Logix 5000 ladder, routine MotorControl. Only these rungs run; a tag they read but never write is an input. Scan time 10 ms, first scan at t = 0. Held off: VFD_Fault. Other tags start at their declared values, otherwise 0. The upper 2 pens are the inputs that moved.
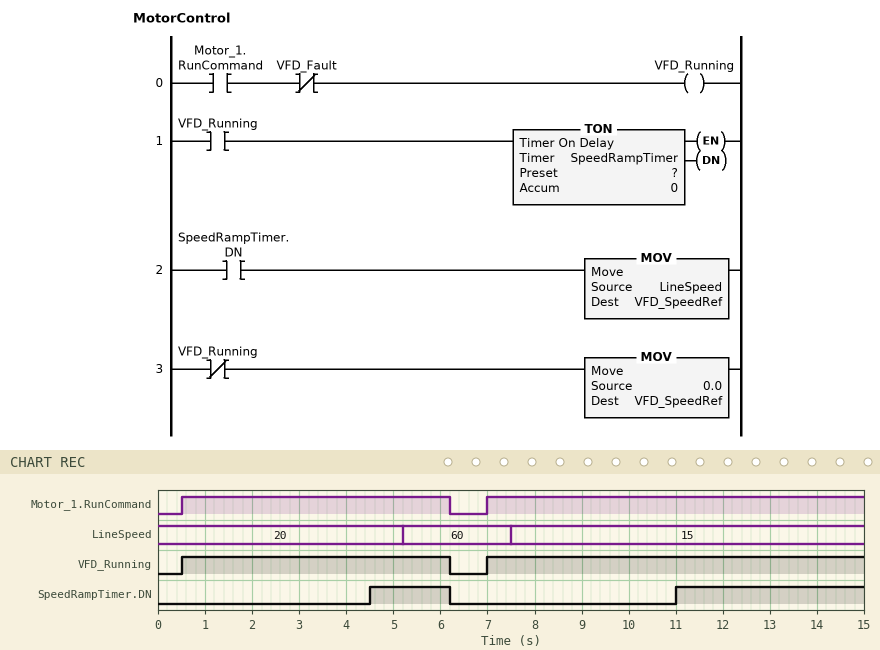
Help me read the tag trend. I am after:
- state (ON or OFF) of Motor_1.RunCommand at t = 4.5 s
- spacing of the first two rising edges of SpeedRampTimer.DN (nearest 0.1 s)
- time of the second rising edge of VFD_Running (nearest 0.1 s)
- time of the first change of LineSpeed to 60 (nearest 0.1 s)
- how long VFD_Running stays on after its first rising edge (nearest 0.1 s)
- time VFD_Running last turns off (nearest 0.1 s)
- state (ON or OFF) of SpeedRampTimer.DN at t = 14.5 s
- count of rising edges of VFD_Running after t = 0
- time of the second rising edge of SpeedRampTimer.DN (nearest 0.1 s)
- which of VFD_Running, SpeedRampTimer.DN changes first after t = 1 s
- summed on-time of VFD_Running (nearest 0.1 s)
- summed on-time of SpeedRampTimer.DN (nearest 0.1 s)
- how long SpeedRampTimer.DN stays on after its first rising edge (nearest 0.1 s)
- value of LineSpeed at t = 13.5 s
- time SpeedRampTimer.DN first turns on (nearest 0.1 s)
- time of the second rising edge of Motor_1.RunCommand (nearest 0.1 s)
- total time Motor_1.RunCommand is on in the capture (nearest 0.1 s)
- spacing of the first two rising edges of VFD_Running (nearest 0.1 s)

ON
6.5 s
7.0 s
5.2 s
5.7 s
6.2 s
ON
2
11.0 s
SpeedRampTimer.DN
13.7 s
5.7 s
1.7 s
15
4.5 s
7.0 s
13.7 s
6.5 s
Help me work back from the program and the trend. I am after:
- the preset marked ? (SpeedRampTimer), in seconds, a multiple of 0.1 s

4.0 s
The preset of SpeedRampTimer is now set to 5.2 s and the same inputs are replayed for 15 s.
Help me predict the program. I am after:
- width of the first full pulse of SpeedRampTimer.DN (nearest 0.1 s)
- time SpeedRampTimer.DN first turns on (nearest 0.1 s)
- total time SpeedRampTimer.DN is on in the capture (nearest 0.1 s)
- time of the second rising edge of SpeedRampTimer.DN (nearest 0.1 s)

0.5 s
5.7 s
3.3 s
12.2 s
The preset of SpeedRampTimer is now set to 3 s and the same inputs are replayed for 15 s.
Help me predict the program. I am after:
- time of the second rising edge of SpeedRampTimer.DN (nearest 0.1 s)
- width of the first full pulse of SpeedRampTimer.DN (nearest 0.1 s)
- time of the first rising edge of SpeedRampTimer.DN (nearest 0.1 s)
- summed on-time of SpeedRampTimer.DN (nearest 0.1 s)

10.0 s
2.7 s
3.5 s
7.7 s
